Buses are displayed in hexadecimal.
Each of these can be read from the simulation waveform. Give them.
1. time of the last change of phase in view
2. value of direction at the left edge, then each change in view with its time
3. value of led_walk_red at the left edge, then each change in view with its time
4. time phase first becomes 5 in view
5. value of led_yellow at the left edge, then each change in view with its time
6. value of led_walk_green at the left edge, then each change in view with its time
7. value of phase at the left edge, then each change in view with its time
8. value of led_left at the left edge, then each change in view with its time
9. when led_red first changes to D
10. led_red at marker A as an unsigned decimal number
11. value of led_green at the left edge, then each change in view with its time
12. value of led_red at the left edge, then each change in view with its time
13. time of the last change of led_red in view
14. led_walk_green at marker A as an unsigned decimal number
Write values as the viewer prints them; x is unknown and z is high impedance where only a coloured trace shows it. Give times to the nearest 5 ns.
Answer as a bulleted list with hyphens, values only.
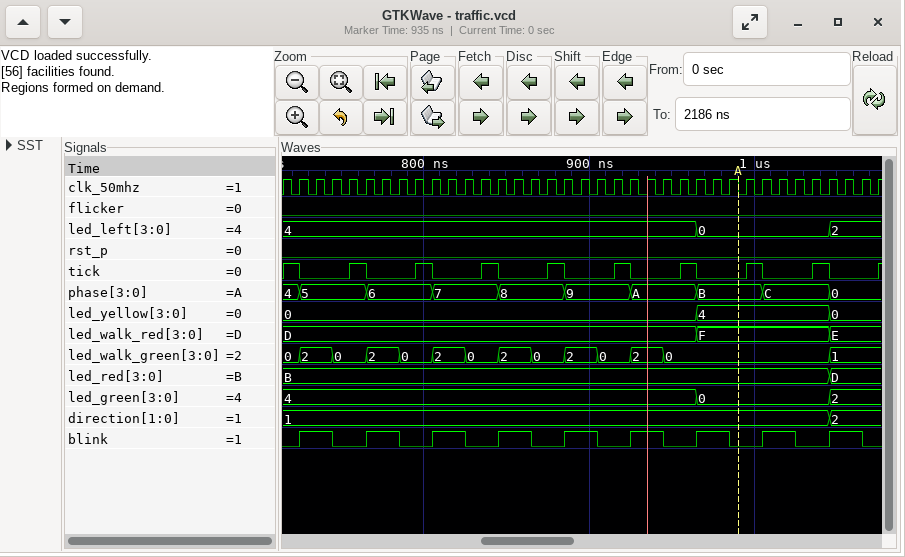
- 1045 ns
- 1, 2 at 1045 ns
- D, F at 965 ns, E at 1045 ns
- 725 ns
- 0, 4 at 965 ns, 0 at 1045 ns
- 0, 2 at 725 ns, 0 at 745 ns, 2 at 765 ns, 0 at 785 ns, 2 at 805 ns, 0 at 825 ns, 2 at 845 ns, 0 at 865 ns, 2 at 885 ns, 0 at 905 ns, 2 at 925 ns, 0 at 945 ns, 1 at 1045 ns
- 4, 5 at 725 ns, 6 at 765 ns, 7 at 805 ns, 8 at 845 ns, 9 at 885 ns, A at 925 ns, B at 965 ns, C at 1005 ns, 0 at 1045 ns
- 4, 0 at 965 ns, 2 at 1045 ns
- 1045 ns
- 11
- 4, 0 at 965 ns, 2 at 1045 ns
- B, D at 1045 ns
- 1045 ns
- 0
